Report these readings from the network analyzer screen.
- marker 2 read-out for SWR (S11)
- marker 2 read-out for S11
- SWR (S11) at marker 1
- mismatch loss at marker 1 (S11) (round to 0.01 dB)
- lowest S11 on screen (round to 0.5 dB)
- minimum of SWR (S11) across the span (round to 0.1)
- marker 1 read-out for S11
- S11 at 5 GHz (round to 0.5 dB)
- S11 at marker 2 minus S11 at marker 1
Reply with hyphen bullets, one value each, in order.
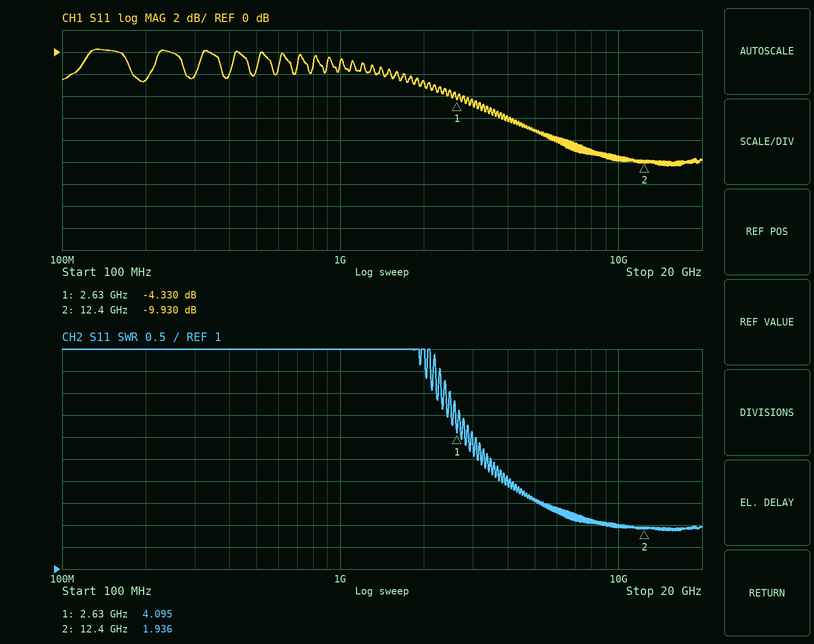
- 1.936
- -9.930 dB
- 4.095
- 2.00 dB
- -10.5 dB
- 1.9
- -4.330 dB
- -7.0 dB
- -5.600 dB
